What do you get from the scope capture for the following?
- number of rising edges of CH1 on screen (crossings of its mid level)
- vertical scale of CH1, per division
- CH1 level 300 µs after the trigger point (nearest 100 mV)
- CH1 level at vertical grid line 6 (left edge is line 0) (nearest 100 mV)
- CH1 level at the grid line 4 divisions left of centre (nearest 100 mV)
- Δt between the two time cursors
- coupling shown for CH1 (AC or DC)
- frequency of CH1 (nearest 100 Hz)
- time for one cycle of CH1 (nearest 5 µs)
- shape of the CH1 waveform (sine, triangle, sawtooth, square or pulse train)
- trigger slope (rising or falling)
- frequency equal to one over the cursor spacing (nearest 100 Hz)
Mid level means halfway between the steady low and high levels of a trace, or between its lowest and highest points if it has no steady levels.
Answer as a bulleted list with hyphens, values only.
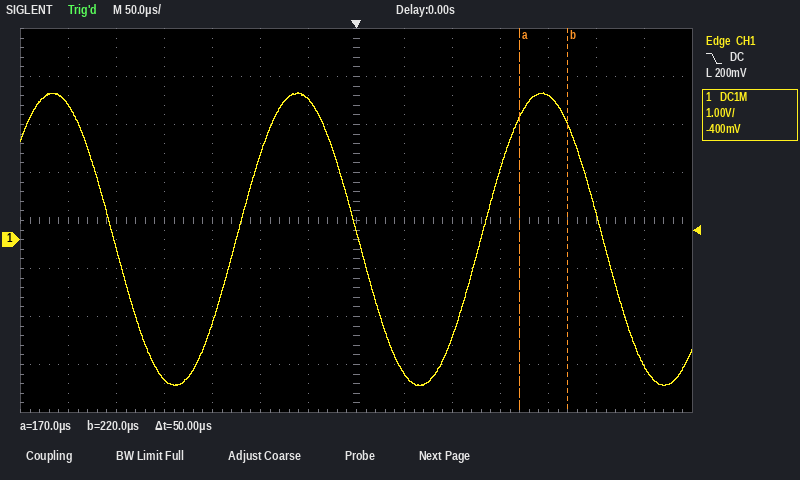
- 2
- 1 V
- -2.6 V
- 2.9 V
- -2.9 V
- 50 µs
- DC
- 3.9 kHz
- 255 µs
- sine
- falling
- 20.0 kHz
